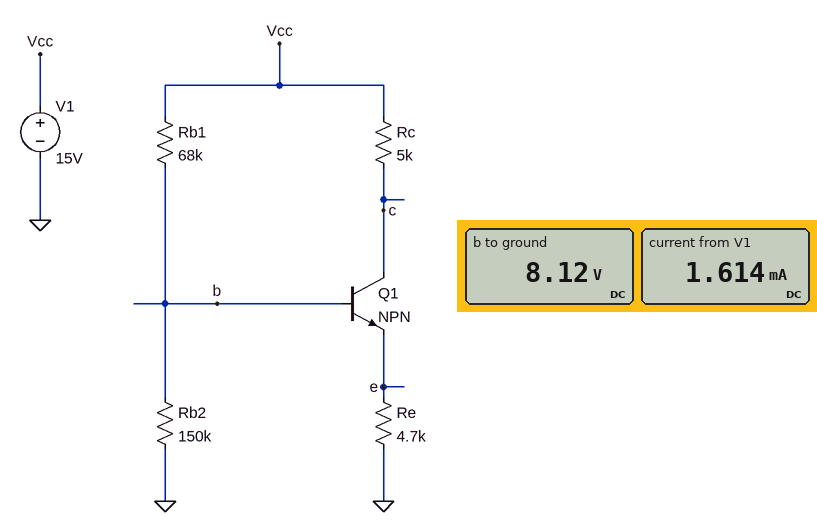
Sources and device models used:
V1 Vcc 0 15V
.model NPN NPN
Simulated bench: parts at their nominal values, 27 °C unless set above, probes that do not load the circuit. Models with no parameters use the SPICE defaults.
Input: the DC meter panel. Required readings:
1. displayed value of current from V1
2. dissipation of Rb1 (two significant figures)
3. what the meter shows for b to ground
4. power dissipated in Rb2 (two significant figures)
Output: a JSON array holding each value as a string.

["1.614 mA", "700 µW", "8.12 V", "440 µW"]
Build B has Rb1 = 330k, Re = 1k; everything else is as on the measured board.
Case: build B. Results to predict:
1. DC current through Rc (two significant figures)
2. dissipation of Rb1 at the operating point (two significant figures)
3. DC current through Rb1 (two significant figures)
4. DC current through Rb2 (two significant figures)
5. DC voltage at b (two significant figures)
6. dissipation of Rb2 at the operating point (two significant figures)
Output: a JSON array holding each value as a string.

["1.9 mA", "460 µW", "37 µA", "18 µA", "2.7 V", "49 µW"]
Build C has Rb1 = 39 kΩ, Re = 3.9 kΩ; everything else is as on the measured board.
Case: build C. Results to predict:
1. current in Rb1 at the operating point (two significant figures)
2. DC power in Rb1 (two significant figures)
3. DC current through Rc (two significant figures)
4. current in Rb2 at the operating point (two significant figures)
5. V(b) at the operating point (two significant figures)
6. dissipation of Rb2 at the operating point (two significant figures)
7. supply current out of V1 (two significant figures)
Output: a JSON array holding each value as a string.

["190 µA", "1.4 mW", "1.6 mA", "51 µA", "7.6 V", "390 µW", "1.8 mA"]
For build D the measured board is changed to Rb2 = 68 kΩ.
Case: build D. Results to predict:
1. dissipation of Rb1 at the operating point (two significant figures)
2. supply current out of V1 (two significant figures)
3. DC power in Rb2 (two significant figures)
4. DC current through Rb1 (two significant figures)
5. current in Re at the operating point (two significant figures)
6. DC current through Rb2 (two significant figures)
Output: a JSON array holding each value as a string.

["930 µW", "1.4 mA", "730 µW", "120 µA", "1.3 mA", "100 µA"]
